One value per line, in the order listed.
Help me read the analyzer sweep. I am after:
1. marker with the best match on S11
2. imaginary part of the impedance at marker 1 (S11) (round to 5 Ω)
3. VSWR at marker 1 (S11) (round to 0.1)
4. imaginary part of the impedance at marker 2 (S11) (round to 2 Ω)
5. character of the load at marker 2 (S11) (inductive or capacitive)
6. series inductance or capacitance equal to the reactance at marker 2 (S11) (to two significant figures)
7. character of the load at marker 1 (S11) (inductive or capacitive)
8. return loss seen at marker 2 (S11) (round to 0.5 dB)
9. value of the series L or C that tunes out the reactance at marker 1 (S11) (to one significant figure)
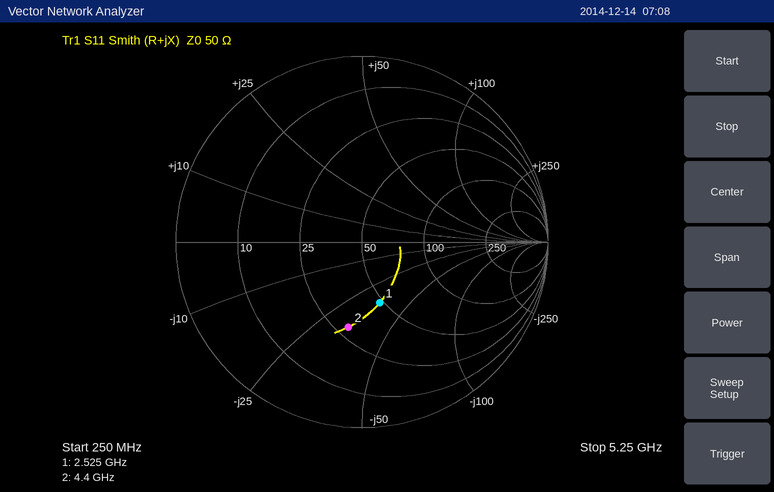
marker 1
-35 Ω
2.0
-34 Ω
capacitive
1.1 pF
capacitive
6.5 dB
2 nH
